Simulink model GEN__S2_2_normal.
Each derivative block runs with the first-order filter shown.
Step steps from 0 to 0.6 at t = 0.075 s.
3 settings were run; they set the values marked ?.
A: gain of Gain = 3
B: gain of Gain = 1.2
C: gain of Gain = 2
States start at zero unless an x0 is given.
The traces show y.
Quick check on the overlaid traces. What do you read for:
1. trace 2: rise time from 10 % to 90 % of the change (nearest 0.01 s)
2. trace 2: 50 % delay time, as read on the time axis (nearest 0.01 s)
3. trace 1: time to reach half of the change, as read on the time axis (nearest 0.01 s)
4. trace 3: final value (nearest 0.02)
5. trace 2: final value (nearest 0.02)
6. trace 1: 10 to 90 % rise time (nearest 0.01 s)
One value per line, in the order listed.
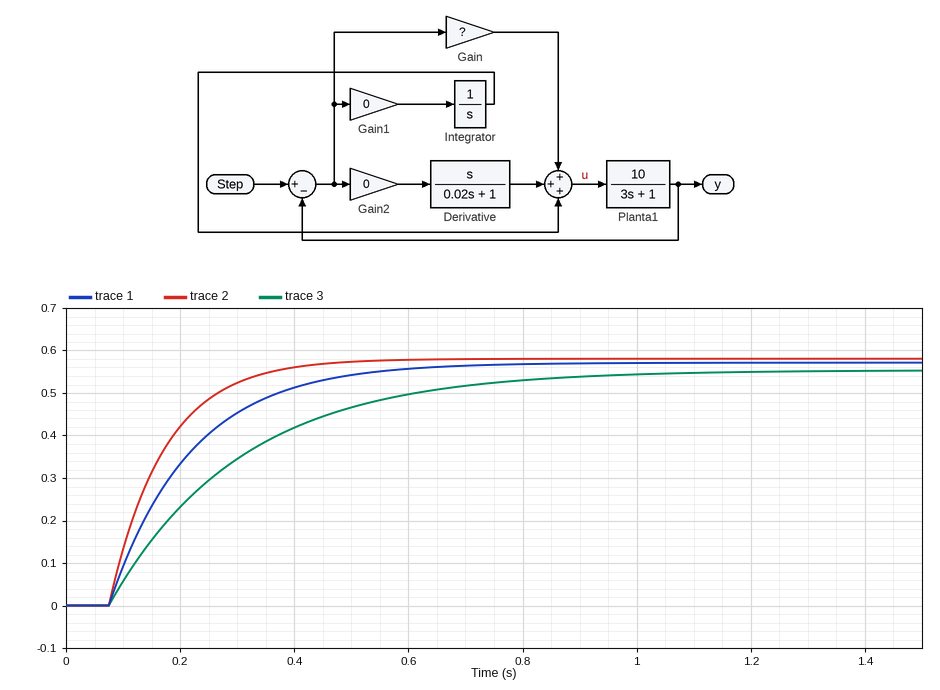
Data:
0.21 s
0.14 s
0.17 s
0.56
0.58
0.31 s
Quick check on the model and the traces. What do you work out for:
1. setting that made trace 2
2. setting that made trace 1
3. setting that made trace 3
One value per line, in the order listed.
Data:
A
C
B
